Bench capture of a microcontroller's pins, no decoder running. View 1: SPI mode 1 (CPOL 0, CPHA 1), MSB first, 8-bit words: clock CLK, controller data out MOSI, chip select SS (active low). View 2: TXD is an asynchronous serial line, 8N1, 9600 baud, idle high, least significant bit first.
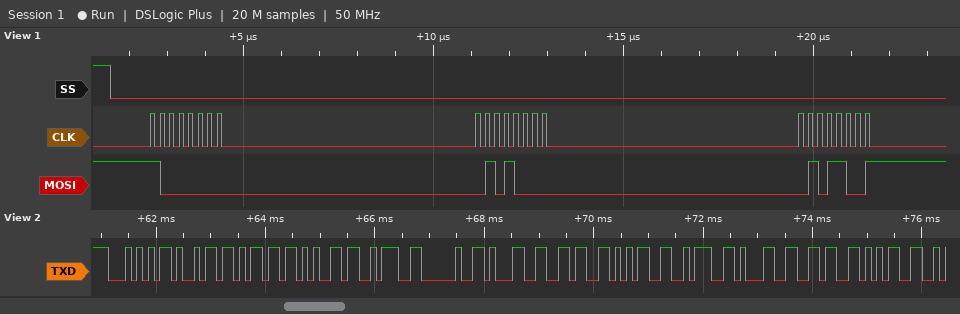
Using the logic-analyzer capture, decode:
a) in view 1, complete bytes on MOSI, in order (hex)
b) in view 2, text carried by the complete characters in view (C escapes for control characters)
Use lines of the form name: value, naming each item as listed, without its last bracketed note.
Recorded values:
in view 1, complete bytes on MOSI, in order: 80 50 59
in view 2, text carried by the complete characters in view: "Time: 165:165"
